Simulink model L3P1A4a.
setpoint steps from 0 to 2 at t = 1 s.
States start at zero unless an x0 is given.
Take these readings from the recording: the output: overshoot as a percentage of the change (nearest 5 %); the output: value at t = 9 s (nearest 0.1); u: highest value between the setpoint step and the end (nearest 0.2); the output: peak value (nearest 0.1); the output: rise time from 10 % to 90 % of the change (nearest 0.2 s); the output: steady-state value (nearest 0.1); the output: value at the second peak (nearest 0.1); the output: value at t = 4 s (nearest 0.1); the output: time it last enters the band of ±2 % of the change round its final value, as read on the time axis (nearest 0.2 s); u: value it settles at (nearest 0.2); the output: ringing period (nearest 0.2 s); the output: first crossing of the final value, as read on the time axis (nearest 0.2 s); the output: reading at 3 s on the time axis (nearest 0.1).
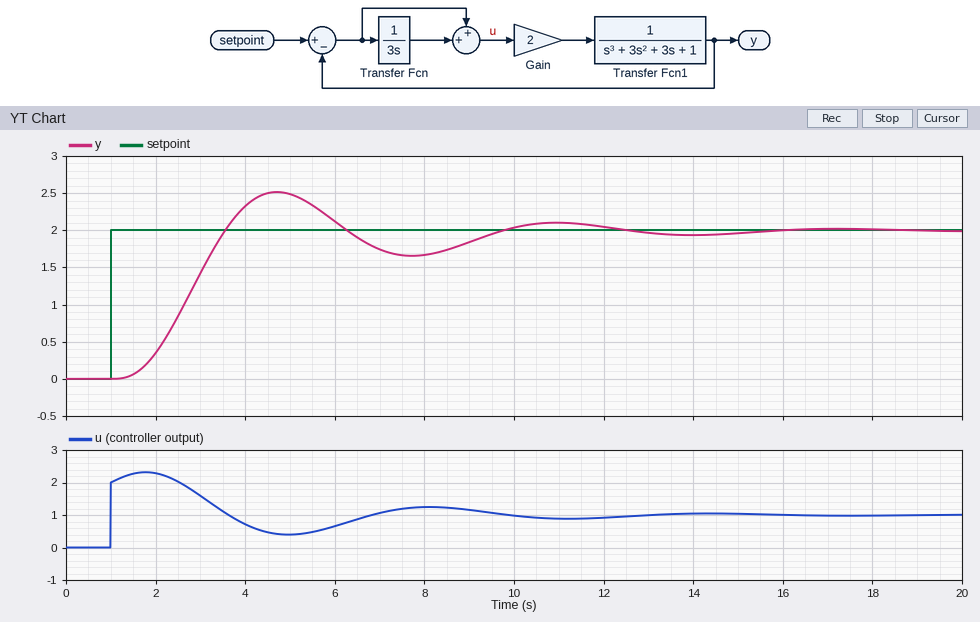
25 %
1.8
2.4
2.5
1.6 s
2.0
2.1
2.3
15.0 s
1.0
6.2 s
3.6 s
1.4
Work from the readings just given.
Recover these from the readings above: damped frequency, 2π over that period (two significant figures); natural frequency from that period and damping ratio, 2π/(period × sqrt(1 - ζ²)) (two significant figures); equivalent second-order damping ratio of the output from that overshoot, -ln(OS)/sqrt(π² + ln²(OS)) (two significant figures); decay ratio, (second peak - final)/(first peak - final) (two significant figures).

1.0 rad/s
1.1 rad/s
0.40
0.20
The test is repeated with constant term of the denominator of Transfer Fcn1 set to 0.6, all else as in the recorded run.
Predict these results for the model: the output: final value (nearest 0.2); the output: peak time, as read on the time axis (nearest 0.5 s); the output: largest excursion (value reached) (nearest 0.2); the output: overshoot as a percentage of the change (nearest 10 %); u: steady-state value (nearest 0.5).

2.0
5.0 s
2.8
40 %
0.5
